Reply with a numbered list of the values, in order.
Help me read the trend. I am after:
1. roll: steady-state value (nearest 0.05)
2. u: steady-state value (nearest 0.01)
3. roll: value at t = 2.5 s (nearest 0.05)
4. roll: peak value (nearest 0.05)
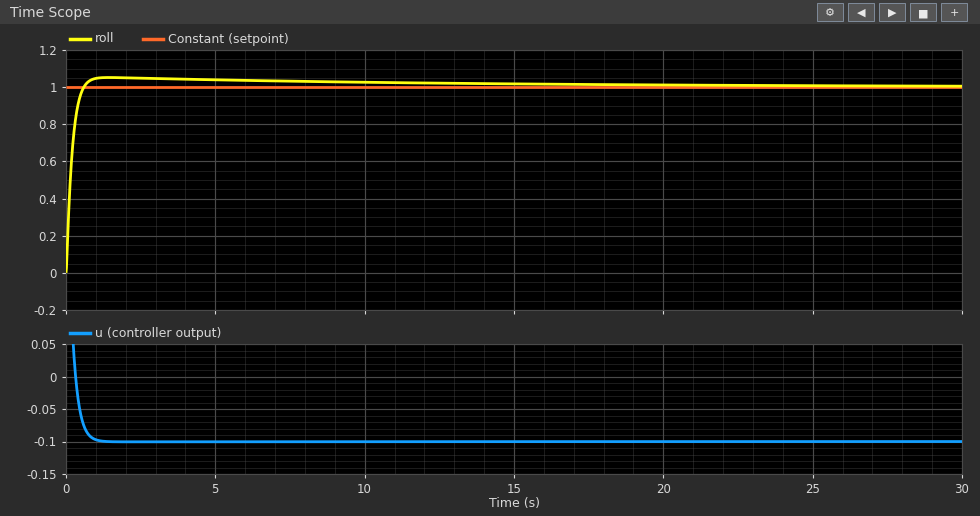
1. 1.00
2. -0.10
3. 1.05
4. 1.05
